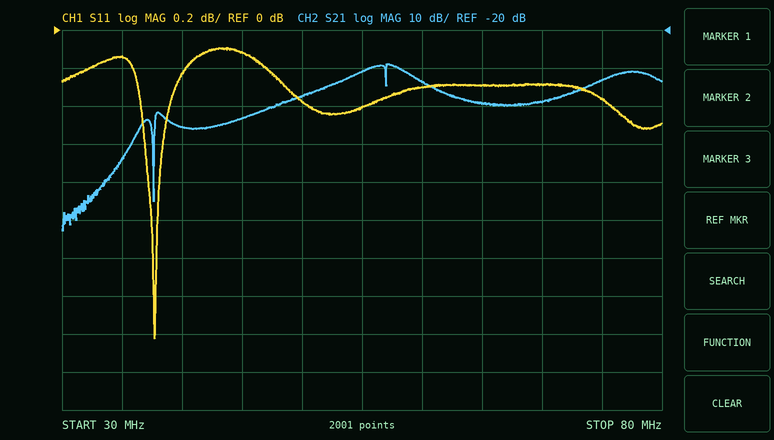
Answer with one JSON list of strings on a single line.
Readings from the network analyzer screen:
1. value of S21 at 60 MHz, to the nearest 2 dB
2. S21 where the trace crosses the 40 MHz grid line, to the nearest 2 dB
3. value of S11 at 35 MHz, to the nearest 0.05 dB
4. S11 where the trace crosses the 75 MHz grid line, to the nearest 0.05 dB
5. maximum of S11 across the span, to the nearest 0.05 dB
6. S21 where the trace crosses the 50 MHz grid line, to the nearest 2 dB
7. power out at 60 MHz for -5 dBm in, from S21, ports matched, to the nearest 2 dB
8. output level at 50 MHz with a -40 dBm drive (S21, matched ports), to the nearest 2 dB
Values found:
["-34 dB", "-46 dB", "-0.15 dB", "-0.35 dB", "-0.10 dB", "-38 dB", "-38 dBm", "-78 dBm"]
